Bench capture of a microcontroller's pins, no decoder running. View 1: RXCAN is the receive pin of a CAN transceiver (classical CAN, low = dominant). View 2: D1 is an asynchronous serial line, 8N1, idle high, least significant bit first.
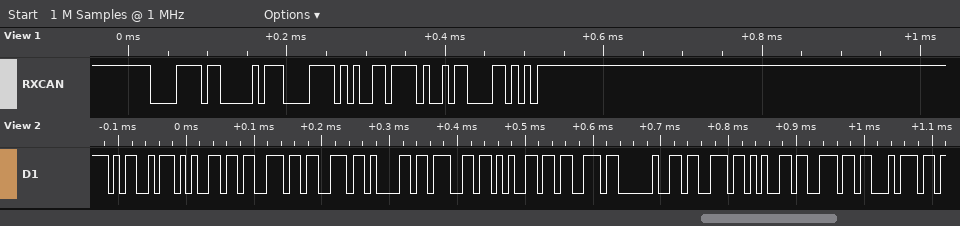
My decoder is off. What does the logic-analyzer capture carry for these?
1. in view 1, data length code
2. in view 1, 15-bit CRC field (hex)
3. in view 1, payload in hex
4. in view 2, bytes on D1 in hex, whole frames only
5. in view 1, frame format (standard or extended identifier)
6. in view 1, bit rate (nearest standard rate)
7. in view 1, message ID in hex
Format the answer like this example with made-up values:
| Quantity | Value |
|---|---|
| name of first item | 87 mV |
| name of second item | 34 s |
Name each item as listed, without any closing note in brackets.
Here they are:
| Quantity | Value |
|---|---|
| in view 1, data length code | 3 |
| in view 1, 15-bit CRC field | 0x161A |
| in view 1, payload in hex | 87 A9 BD |
| in view 2, bytes on D1 in hex, whole frames only | 4D 65 73 73 61 67 65 73 20 73 65 6E 74 |
| in view 1, frame format | standard |
| in view 1, bit rate | 125 kbit/s |
| in view 1, message ID in hex | 0x0F6 |
